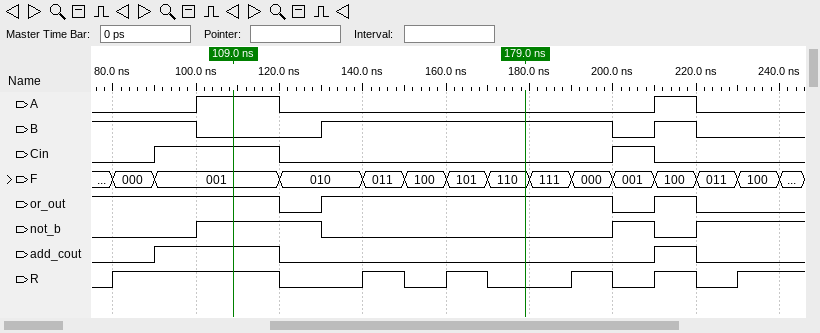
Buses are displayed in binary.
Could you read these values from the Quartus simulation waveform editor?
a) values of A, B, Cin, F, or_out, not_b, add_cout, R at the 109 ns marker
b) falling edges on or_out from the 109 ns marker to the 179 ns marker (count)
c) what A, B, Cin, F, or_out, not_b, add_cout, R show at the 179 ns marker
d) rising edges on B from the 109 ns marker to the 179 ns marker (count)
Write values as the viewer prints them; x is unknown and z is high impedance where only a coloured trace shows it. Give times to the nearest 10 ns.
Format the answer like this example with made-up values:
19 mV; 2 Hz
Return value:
A=1, B=0, Cin=1, F=001, or_out=1, not_b=1, add_cout=1, R=1; 1; A=0, B=1, Cin=0, F=110, or_out=1, not_b=0, add_cout=0, R=0; 1
